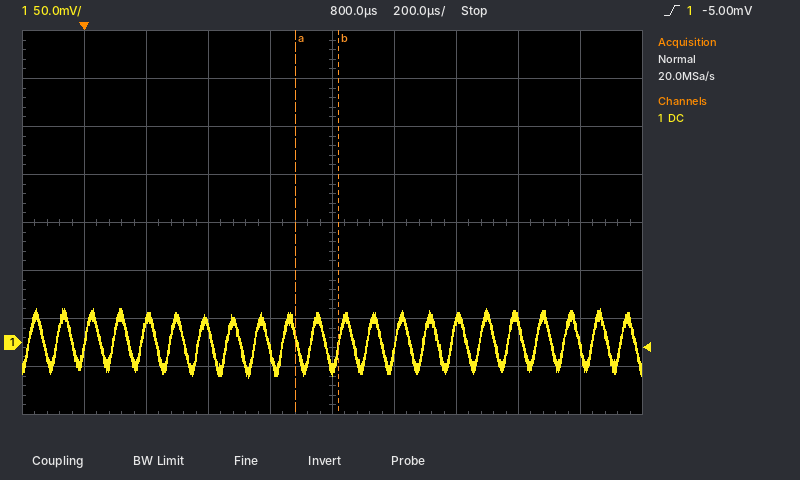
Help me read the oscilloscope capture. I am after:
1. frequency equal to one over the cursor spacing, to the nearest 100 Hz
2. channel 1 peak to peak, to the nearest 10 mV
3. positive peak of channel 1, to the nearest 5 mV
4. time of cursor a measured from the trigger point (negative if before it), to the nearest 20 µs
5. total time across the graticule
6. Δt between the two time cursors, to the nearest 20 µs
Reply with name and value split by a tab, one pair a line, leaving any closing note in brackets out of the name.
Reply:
frequency equal to one over the cursor spacing, to the nearest 100 Hz	7.1 kHz
channel 1 peak to peak, to the nearest 10 mV	70 mV
positive peak of channel 1, to the nearest 5 mV	35 mV
time of cursor a measured from the trigger point (negative if before it), to the nearest 20 µs	+680 µs
total time across the graticule	2 ms
Δt between the two time cursors, to the nearest 20 µs	140 µs
